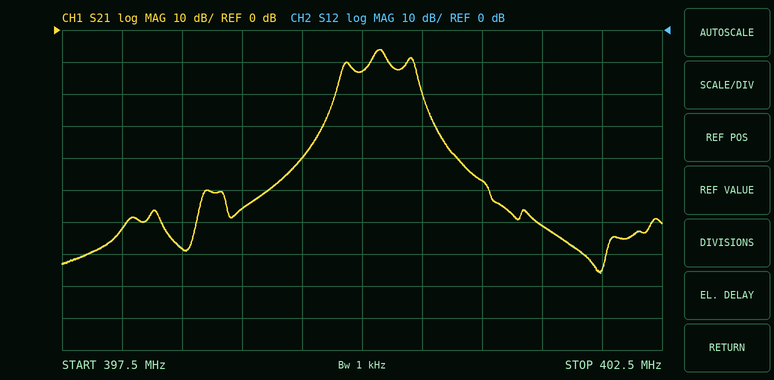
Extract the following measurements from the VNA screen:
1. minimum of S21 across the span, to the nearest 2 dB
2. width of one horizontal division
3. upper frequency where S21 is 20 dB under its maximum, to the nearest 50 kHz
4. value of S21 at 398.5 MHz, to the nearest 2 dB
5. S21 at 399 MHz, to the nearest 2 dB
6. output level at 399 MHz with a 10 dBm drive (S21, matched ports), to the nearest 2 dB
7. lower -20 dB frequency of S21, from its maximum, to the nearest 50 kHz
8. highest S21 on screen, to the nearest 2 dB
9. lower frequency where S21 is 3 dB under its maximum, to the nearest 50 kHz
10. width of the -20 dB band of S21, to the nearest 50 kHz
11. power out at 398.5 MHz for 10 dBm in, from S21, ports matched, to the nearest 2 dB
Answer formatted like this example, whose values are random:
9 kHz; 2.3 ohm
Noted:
-76 dB; 500 kHz; 400.55 MHz; -68 dB; -56 dB; -46 dBm; 399.70 MHz; -6 dB; 400.10 MHz; 850 kHz; -58 dBm
